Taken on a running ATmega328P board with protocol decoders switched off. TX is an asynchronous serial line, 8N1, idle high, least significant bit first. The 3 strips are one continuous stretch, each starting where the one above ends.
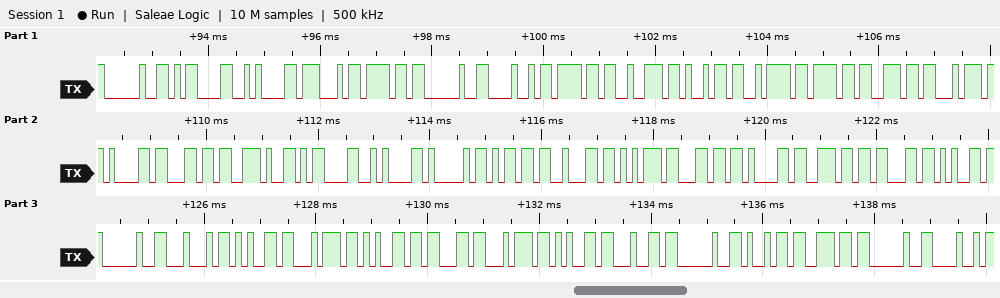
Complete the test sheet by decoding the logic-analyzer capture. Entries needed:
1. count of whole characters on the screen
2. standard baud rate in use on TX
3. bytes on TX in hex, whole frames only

42
9600 baud
20 0D 0A 47 6F 20 48 6F 72 69 7A 6F 6E 74 61 6C 2E 0D 0A 41 6D 62 75 6C 61 6E 63 65 20 44 65 74 65 63 74 65 64 20 69 6E 20 48
